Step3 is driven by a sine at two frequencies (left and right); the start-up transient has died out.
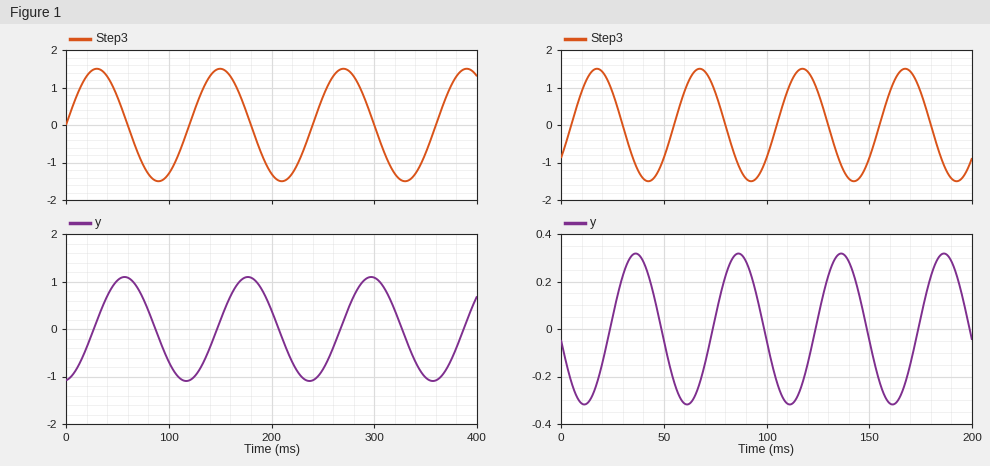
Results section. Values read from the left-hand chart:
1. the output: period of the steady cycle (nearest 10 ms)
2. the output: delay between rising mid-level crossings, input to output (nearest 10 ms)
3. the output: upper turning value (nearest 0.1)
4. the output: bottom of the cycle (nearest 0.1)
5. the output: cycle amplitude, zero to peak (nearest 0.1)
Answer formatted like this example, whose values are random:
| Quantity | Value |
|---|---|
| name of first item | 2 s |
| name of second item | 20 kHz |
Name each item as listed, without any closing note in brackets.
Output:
| Quantity | Value |
|---|---|
| the output: period of the steady cycle | 120 ms |
| the output: delay between rising mid-level crossings, input to output | 30 ms |
| the output: upper turning value | 1.1 |
| the output: bottom of the cycle | -1.1 |
| the output: cycle amplitude, zero to peak | 1.1 |
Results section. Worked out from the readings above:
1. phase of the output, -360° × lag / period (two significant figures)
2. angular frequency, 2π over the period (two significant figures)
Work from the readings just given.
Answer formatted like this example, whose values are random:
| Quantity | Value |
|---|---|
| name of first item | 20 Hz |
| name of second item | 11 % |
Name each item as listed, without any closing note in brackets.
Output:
| Quantity | Value |
|---|---|
| phase of the output, -360° × lag / period | -90° |
| angular frequency, 2π over the period | 0.052 rad/ms |
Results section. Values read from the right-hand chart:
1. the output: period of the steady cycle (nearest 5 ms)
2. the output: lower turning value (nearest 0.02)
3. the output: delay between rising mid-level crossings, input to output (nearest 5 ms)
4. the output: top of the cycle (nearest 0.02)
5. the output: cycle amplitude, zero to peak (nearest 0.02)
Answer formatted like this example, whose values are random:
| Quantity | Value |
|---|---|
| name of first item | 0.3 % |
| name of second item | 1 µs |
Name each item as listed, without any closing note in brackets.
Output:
| Quantity | Value |
|---|---|
| the output: period of the steady cycle | 50 ms |
| the output: lower turning value | -0.32 |
| the output: delay between rising mid-level crossings, input to output | 20 ms |
| the output: top of the cycle | 0.32 |
| the output: cycle amplitude, zero to peak | 0.32 |
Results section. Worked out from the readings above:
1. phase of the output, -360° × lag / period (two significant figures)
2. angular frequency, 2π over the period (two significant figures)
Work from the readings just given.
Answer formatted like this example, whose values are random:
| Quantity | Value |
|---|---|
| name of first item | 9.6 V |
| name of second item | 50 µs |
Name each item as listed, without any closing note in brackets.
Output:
| Quantity | Value |
|---|---|
| phase of the output, -360° × lag / period | -140° |
| angular frequency, 2π over the period | 0.13 rad/ms |
